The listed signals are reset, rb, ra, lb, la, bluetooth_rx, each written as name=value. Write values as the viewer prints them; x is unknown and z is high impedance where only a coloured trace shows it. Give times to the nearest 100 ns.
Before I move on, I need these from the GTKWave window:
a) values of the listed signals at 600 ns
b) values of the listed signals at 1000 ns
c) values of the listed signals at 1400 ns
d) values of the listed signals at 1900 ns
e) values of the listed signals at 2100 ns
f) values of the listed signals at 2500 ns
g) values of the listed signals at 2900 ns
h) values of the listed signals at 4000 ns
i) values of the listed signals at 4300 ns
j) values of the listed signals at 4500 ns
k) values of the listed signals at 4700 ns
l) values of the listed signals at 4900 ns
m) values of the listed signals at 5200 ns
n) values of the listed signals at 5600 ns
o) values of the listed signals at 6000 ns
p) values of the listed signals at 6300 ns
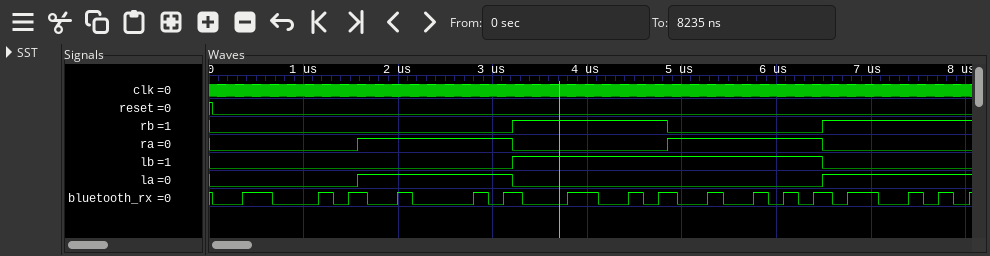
reset=0, rb=0, ra=0, lb=0, la=0, bluetooth_rx=1
reset=0, rb=0, ra=0, lb=0, la=0, bluetooth_rx=0
reset=0, rb=0, ra=0, lb=0, la=0, bluetooth_rx=0
reset=0, rb=0, ra=1, lb=0, la=1, bluetooth_rx=0
reset=0, rb=0, ra=1, lb=0, la=1, bluetooth_rx=1
reset=0, rb=0, ra=1, lb=0, la=1, bluetooth_rx=0
reset=0, rb=0, ra=1, lb=0, la=1, bluetooth_rx=1
reset=0, rb=1, ra=0, lb=1, la=0, bluetooth_rx=1
reset=0, rb=1, ra=0, lb=1, la=0, bluetooth_rx=0
reset=0, rb=1, ra=0, lb=1, la=0, bluetooth_rx=1
reset=0, rb=1, ra=0, lb=1, la=0, bluetooth_rx=0
reset=0, rb=0, ra=1, lb=1, la=0, bluetooth_rx=1
reset=0, rb=0, ra=1, lb=1, la=0, bluetooth_rx=0
reset=0, rb=0, ra=1, lb=1, la=0, bluetooth_rx=0
reset=0, rb=0, ra=1, lb=1, la=0, bluetooth_rx=0
reset=0, rb=0, ra=1, lb=1, la=0, bluetooth_rx=0
